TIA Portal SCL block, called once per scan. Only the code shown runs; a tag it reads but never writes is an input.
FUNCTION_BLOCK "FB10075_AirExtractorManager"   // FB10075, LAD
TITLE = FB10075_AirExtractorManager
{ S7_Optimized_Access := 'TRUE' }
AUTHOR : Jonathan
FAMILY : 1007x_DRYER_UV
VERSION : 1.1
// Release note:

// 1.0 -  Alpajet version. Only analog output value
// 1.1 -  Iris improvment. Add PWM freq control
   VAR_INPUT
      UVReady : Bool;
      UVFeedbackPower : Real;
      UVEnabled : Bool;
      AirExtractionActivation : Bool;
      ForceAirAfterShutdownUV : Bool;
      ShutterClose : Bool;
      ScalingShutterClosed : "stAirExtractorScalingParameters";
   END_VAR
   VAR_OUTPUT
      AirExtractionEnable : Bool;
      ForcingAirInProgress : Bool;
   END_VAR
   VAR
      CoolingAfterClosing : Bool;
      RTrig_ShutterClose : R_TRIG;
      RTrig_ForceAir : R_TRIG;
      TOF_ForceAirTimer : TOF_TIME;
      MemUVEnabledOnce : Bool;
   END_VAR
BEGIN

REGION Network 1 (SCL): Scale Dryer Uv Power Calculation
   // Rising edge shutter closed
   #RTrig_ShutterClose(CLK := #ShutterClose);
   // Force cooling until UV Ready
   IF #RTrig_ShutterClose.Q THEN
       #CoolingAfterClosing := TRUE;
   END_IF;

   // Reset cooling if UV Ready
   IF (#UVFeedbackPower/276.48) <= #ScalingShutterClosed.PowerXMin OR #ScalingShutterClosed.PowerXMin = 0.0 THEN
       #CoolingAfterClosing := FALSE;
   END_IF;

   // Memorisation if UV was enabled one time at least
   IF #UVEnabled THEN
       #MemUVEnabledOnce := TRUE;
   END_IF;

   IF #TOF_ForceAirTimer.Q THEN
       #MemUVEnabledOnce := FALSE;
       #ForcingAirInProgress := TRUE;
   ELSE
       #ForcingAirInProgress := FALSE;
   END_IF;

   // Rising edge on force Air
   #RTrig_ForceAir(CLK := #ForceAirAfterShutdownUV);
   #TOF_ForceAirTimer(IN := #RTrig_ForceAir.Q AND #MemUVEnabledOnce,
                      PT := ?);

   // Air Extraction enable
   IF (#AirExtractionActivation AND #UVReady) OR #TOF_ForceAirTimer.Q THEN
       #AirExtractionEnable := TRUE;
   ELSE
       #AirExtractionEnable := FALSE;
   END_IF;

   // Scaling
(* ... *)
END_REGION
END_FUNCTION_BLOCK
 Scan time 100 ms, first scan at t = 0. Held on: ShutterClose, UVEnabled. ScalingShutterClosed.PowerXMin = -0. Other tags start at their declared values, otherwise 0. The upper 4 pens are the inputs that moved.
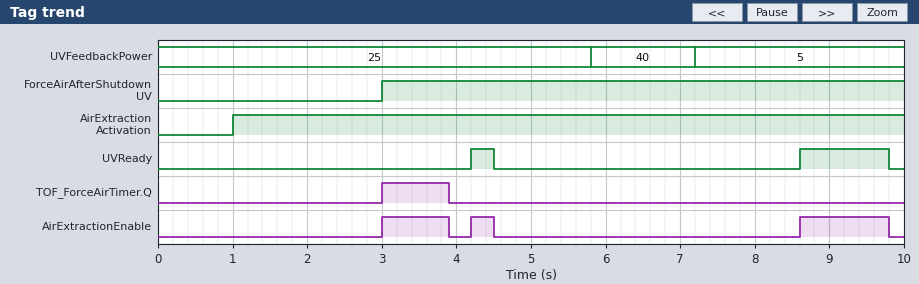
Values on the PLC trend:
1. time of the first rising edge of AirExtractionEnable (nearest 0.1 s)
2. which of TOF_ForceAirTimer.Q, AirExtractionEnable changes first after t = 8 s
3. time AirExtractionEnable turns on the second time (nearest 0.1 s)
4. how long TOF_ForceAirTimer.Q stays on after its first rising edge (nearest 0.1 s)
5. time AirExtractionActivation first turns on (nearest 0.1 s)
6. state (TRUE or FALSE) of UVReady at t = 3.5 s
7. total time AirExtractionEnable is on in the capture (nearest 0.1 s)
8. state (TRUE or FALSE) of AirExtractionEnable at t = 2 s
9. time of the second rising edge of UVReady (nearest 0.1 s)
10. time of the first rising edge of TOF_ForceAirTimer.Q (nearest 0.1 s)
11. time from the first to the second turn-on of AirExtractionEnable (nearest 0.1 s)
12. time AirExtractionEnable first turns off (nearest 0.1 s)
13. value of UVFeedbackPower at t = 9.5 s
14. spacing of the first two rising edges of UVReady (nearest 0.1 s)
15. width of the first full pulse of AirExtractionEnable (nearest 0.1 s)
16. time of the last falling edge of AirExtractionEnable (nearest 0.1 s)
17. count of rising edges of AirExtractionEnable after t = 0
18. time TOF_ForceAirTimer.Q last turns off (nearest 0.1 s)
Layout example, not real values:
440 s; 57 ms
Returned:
3.0 s; AirExtractionEnable; 4.2 s; 0.9 s; 1.0 s; FALSE; 2.4 s; FALSE; 8.6 s; 3.0 s; 1.2 s; 3.9 s; 5; 4.4 s; 0.9 s; 9.8 s; 3; 3.9 s
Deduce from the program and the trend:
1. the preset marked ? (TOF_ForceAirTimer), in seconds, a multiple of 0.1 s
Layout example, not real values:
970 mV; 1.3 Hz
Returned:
0.8 s
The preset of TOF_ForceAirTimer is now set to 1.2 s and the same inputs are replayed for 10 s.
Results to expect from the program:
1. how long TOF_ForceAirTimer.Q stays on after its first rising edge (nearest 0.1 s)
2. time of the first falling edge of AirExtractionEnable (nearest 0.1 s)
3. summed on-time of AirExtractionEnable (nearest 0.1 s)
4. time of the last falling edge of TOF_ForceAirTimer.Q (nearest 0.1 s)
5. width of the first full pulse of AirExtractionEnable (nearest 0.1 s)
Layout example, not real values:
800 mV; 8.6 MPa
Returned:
1.3 s; 4.5 s; 2.7 s; 4.3 s; 1.5 s
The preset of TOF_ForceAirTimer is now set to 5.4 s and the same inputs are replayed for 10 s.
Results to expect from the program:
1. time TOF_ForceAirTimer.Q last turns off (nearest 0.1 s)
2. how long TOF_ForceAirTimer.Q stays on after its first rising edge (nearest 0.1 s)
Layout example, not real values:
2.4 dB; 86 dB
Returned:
8.5 s; 5.5 s
